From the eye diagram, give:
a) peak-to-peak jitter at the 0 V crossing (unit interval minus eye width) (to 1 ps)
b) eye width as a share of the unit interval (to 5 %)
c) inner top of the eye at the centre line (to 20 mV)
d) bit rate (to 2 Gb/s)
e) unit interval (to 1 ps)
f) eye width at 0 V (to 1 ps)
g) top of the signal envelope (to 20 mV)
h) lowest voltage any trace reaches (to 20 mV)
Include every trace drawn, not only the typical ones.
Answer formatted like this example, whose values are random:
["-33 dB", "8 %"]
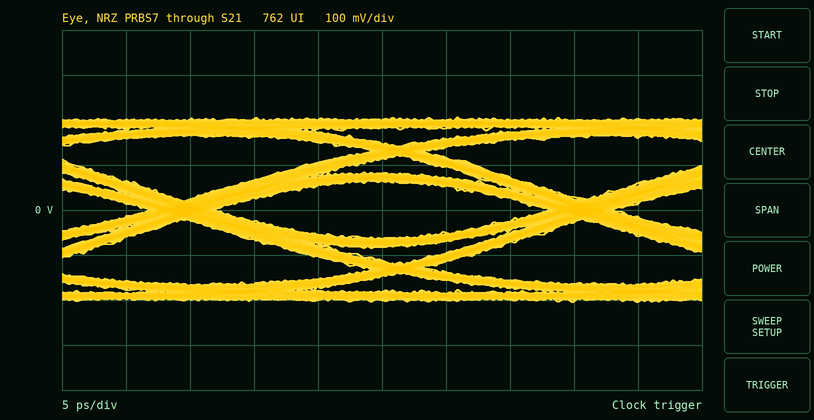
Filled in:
["5 ps", "85 %", "60 mV", "32 Gb/s", "31 ps", "26 ps", "200 mV", "-200 mV"]
